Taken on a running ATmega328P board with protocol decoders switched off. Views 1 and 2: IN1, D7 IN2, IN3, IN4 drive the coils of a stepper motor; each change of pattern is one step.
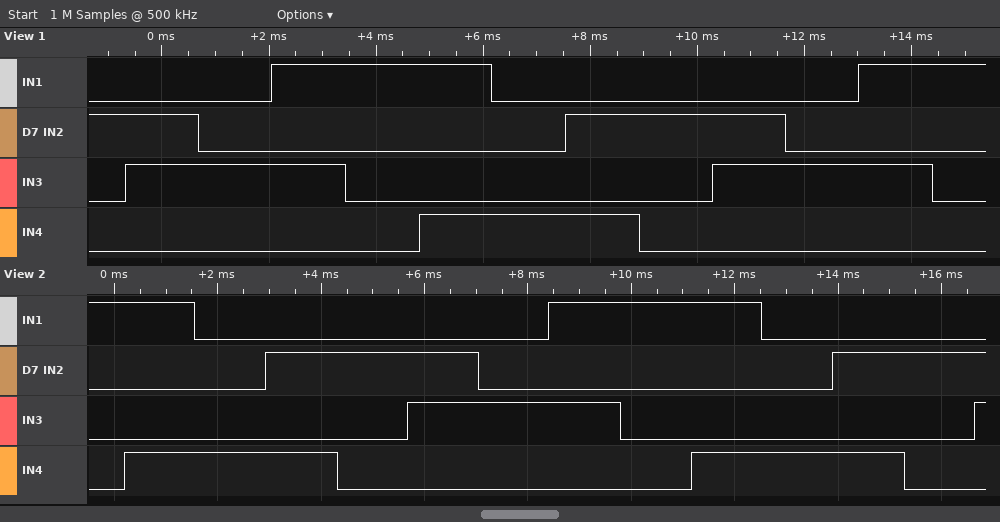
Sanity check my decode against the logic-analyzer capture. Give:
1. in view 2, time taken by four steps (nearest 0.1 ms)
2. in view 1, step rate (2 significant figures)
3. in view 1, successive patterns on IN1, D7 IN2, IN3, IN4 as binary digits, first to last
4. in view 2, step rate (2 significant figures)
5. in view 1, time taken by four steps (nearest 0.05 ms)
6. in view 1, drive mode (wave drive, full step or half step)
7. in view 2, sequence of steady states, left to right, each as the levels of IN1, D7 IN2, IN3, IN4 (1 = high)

5.5 ms
730 steps/s
0100 0110 0010 1010 1000 1001 0001 0101 0100 0110 0010 1010 1000
730 steps/s
5.50 ms
half step
1000 1001 0001 0101 0100 0110 0010 1010 1000 1001 0001 0101 0100 0110
